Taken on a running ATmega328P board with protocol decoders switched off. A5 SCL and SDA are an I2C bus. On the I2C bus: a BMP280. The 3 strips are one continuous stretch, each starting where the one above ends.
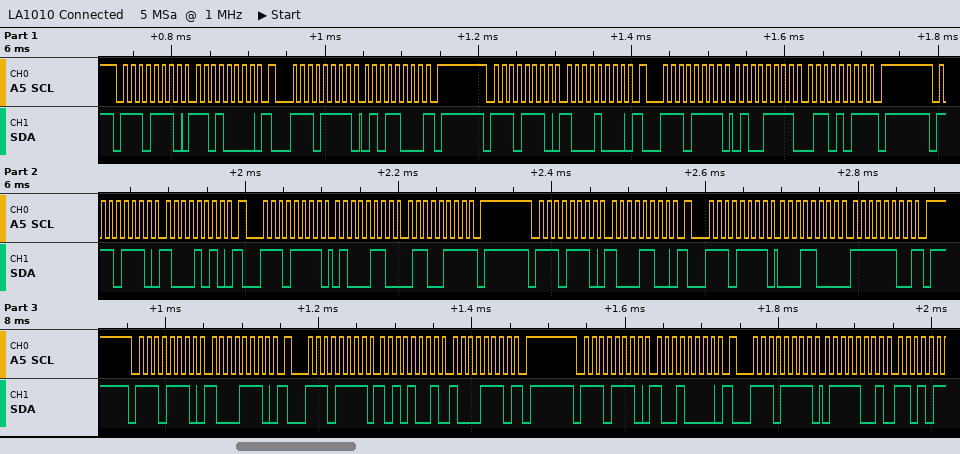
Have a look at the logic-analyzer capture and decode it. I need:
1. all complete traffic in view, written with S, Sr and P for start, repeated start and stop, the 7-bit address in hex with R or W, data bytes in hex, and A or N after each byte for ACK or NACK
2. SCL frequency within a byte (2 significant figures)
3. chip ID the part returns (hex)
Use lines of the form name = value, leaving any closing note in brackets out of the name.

all complete traffic in view, written with S, Sr and P for start, repeated start and stop, the 7-bit address in hex with R or W, data bytes in hex, and A or N after each byte for ACK or NACK = S 77W A D0 A Sr 77R A 58 N P S 77W A 88 A Sr 77R A 4F A 6B N P S 77W A 8A A Sr 77R A 46 A 67 N P S 77W A 8C A Sr 77R A 18 A FC N P S 77W A 8E A Sr 77R A A9 A 8E N P S 77W A 90 A Sr 77R A 79 A
SCL frequency within a byte = 100 kHz
chip ID the part returns = 0x58
